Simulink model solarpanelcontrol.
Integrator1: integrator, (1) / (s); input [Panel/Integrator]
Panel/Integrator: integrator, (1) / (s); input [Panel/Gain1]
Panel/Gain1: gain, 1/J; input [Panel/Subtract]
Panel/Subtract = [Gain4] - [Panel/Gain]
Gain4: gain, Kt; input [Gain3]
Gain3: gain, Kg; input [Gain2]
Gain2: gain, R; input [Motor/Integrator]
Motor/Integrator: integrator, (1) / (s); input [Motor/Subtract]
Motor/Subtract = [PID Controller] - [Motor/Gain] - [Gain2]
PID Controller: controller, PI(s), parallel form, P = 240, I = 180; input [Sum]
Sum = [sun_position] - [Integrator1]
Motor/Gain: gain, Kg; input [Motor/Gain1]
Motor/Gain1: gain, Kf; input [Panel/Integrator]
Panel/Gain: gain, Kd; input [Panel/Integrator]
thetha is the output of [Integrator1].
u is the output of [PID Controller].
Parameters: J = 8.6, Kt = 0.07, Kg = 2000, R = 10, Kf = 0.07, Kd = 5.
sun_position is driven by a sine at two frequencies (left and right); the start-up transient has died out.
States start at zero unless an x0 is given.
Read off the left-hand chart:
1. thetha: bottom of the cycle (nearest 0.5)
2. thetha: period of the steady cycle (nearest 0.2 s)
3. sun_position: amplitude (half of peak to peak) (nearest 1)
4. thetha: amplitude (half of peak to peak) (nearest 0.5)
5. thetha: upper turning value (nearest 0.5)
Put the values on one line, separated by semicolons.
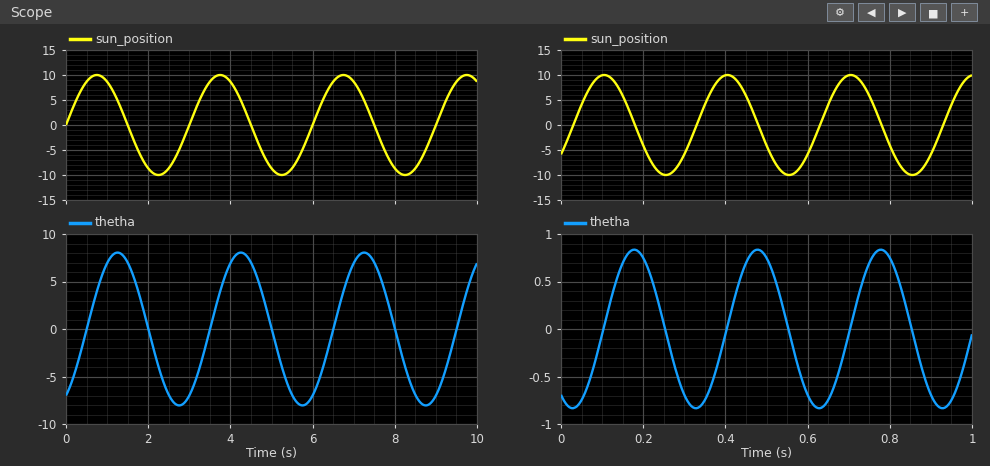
-8.0; 3.0 s; 10; 8.0; 8.0
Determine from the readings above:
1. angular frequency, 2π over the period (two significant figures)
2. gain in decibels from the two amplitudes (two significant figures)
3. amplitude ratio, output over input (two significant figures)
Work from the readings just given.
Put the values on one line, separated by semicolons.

2.1 rad/s; -1.9 dB; 0.80
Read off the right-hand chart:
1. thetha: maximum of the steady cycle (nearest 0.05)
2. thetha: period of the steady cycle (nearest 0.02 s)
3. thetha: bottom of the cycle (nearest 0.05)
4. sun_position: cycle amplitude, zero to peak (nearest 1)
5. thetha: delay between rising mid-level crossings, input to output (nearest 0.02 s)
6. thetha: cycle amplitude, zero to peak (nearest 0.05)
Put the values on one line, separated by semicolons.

0.85; 0.30 s; -0.85; 10; 0.08 s; 0.85
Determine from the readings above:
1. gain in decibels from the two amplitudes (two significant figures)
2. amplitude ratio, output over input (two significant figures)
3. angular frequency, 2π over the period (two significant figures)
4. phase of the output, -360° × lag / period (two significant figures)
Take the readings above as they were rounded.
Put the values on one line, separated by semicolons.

-21 dB; 0.085; 21 rad/s; -96°
